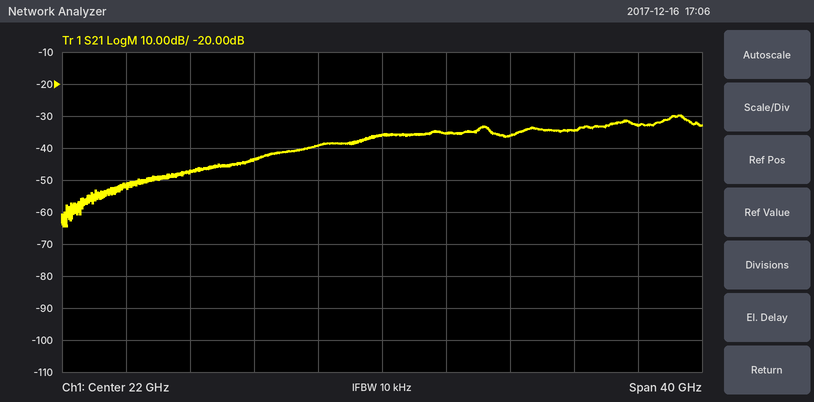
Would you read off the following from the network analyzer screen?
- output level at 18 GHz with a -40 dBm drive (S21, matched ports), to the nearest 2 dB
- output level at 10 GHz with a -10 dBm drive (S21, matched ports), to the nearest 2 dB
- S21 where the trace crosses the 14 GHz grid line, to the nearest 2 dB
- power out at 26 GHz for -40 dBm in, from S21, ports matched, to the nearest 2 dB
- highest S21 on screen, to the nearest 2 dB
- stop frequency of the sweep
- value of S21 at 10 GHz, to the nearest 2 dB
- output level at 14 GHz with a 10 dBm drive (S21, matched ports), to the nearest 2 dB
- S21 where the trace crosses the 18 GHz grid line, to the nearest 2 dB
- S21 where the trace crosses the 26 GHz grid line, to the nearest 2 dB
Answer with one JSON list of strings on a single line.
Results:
["-80 dBm", "-58 dBm", "-44 dB", "-76 dBm", "-30 dB", "42 GHz", "-48 dB", "-34 dBm", "-40 dB", "-36 dB"]
